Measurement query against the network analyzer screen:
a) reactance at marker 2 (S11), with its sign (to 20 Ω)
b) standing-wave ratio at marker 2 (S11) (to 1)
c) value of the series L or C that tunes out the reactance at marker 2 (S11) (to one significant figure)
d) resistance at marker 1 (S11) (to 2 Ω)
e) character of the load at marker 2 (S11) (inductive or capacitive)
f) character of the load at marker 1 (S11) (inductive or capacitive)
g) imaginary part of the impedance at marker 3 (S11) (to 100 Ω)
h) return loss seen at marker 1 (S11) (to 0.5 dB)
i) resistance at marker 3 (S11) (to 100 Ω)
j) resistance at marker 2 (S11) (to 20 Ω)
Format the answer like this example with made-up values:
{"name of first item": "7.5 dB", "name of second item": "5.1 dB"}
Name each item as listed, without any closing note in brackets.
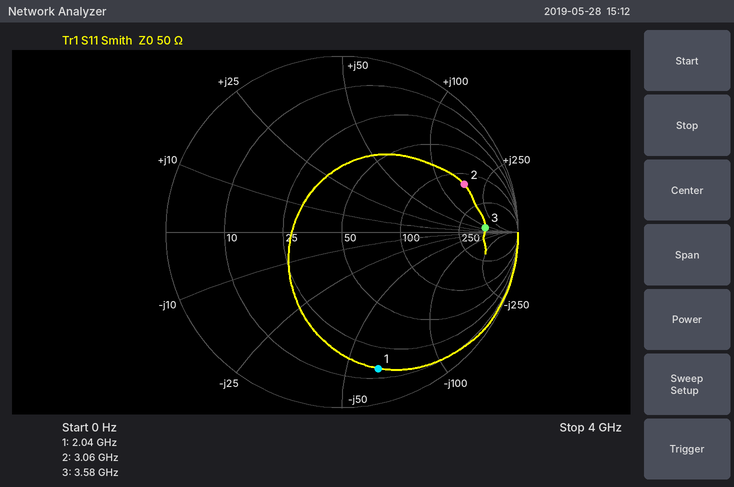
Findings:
{"reactance at marker 2 (S11), with its sign": "+160 Ω", "standing-wave ratio at marker 2 (S11)": "7", "value of the series L or C that tunes out the reactance at marker 2 (S11)": "300 fF", "resistance at marker 1 (S11)": "14 Ω", "character of the load at marker 2 (S11)": "inductive", "character of the load at marker 1 (S11)": "capacitive", "imaginary part of the impedance at marker 3 (S11)": "+100 Ω", "return loss seen at marker 1 (S11)": "2.0 dB", "resistance at marker 3 (S11)": "500 Ω", "resistance at marker 2 (S11)": "140 Ω"}
